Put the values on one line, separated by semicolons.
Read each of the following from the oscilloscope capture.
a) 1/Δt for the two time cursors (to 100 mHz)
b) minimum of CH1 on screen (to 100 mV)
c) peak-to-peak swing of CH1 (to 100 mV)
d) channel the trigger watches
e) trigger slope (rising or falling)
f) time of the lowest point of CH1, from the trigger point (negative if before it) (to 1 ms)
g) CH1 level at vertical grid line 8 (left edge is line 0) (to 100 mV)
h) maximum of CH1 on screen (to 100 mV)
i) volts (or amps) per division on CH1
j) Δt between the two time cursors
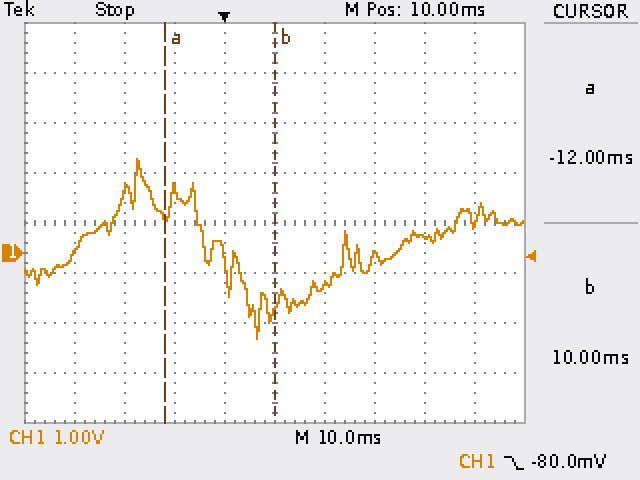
45.5 Hz; -1.7 V; 3.6 V; CH1; falling; +7 ms; 300 mV; 1.9 V; 1 V; 22 ms
